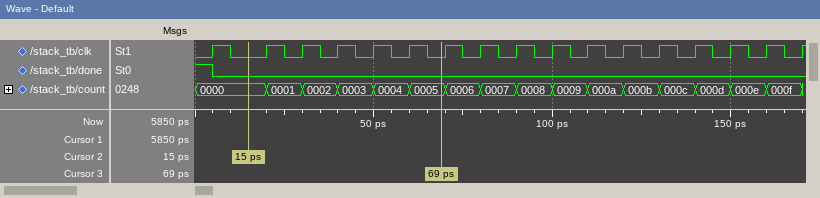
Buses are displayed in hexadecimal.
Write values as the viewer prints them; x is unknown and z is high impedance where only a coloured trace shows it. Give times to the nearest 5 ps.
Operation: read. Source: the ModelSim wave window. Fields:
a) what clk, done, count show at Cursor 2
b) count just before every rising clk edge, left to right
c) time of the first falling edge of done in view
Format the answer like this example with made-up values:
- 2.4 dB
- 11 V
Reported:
- clk=0, done=0, count=0000
- 0000, 0000, 0001, 0002, 0003, 0004, 0005, 0006, 0007, 0008, 0009, 000a, 000b, 000c, 000d, 000e, 000f
- 5 ps
